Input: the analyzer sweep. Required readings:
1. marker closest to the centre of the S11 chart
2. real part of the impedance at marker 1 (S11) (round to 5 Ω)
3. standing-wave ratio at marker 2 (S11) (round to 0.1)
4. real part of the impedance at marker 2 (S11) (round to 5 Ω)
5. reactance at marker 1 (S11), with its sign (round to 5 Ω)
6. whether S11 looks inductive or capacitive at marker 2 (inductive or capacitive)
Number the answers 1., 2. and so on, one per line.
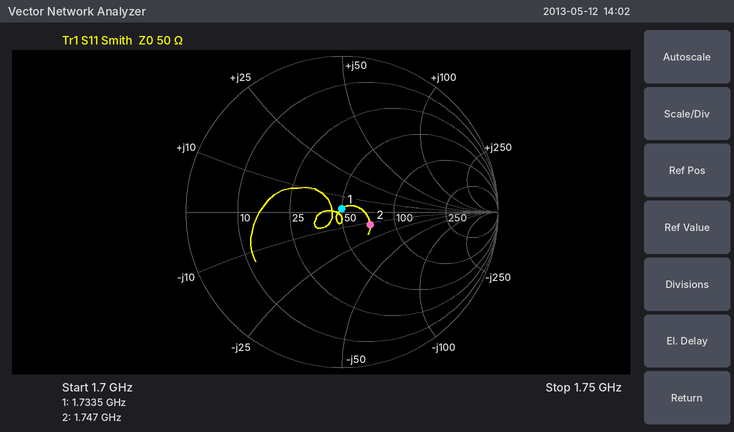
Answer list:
1. marker 1
2. 50 Ω
3. 1.5
4. 70 Ω
5. 0 Ω
6. capacitive
